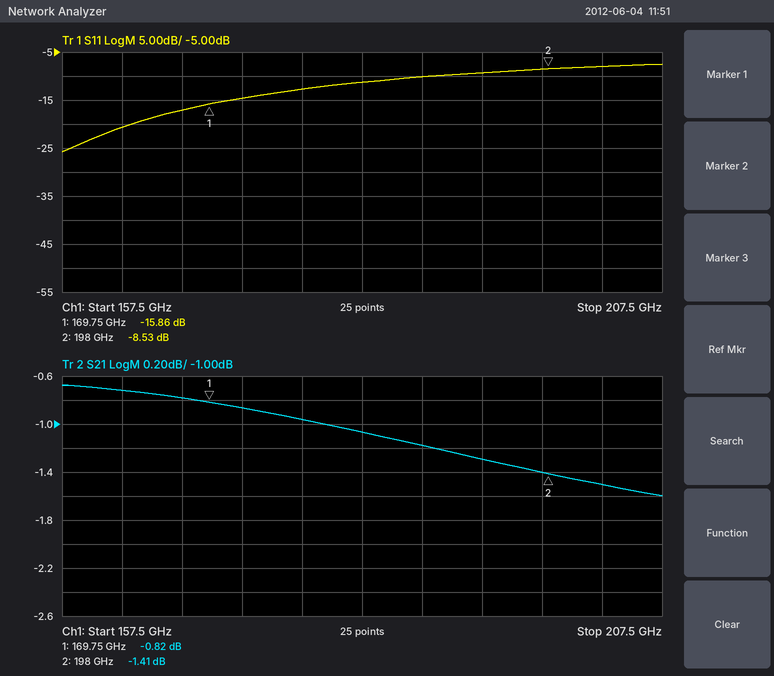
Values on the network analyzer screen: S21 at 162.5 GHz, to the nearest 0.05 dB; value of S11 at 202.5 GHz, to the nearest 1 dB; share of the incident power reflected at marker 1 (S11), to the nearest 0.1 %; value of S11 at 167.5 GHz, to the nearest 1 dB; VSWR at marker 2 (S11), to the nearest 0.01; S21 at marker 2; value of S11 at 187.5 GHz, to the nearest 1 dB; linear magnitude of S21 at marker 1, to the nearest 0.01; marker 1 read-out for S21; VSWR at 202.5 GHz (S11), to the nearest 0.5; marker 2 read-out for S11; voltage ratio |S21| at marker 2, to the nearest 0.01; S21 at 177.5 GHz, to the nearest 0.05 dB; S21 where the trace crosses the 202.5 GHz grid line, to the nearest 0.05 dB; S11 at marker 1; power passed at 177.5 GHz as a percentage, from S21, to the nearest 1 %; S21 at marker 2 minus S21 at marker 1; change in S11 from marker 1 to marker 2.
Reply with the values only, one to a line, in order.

-0.70 dB
-8 dB
2.6 %
-17 dB
2.20
-1.41 dB
-10 dB
0.91
-0.82 dB
2.5
-8.53 dB
0.85
-0.95 dB
-1.50 dB
-15.86 dB
80 %
-0.59 dB
7.33 dB
